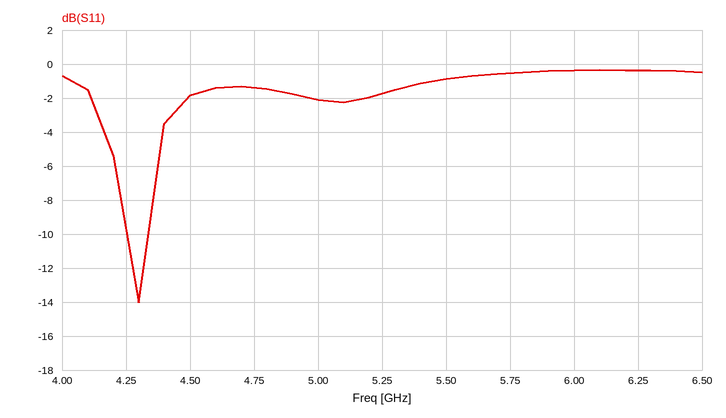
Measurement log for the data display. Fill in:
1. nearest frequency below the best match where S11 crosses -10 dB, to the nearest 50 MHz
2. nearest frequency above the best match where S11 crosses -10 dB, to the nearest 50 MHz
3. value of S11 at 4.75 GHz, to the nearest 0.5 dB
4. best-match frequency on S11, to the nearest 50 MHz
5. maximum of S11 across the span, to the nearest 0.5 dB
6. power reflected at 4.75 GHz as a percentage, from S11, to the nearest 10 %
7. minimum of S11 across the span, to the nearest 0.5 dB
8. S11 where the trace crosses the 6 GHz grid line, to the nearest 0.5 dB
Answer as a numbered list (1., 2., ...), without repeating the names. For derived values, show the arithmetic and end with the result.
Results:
1. 4.25 GHz
2. 4.35 GHz
3. -1.5 dB
4. 4.30 GHz
5. -0.5 dB
6. 10^(-1.5/10) ≈ 70.8 %, so 70 % to the nearest 10 %
7. -14.0 dB
8. -0.5 dB
